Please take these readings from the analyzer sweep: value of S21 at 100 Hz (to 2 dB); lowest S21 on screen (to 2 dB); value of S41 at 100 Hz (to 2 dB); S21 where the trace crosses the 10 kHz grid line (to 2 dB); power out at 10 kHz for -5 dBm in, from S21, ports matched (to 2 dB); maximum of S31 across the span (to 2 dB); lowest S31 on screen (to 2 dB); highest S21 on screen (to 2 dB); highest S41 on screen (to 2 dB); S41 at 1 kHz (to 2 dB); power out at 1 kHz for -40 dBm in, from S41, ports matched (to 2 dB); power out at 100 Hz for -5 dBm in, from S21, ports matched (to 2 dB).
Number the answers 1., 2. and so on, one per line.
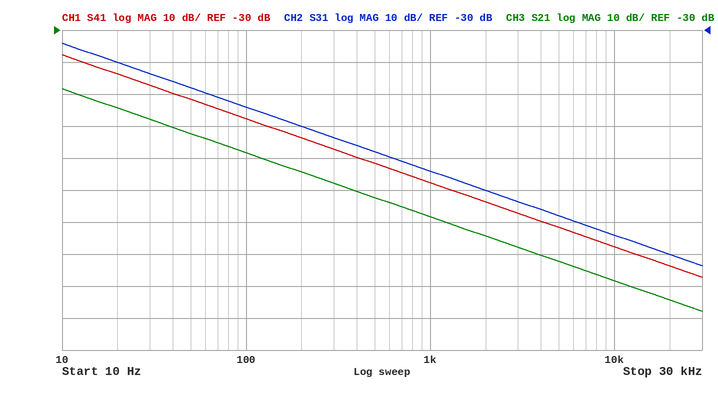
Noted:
1. -68 dB
2. -118 dB
3. -58 dB
4. -108 dB
5. -114 dBm
6. -34 dB
7. -104 dB
8. -48 dB
9. -38 dB
10. -78 dB
11. -118 dBm
12. -74 dBm
